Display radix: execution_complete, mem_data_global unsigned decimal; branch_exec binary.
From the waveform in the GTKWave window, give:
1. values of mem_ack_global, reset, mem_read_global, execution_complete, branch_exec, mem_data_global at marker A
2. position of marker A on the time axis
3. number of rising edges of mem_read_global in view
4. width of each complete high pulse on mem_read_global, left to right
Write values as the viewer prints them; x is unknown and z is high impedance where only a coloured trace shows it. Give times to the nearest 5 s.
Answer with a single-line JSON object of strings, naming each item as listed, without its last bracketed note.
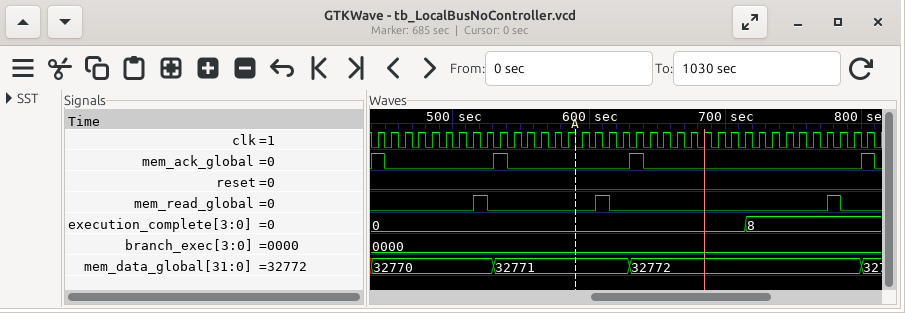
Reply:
{"values of mem_ack_global, reset, mem_read_global, execution_complete, branch_exec, mem_data_global at marker A": "mem_ack_global=0, reset=0, mem_read_global=0, execution_complete=0, branch_exec=0000, mem_data_global=32771", "position of marker A on the time axis": "590 s", "number of rising edges of mem_read_global in view": "3", "width of each complete high pulse on mem_read_global, left to right": "10 s, 10 s, 10 s"}
